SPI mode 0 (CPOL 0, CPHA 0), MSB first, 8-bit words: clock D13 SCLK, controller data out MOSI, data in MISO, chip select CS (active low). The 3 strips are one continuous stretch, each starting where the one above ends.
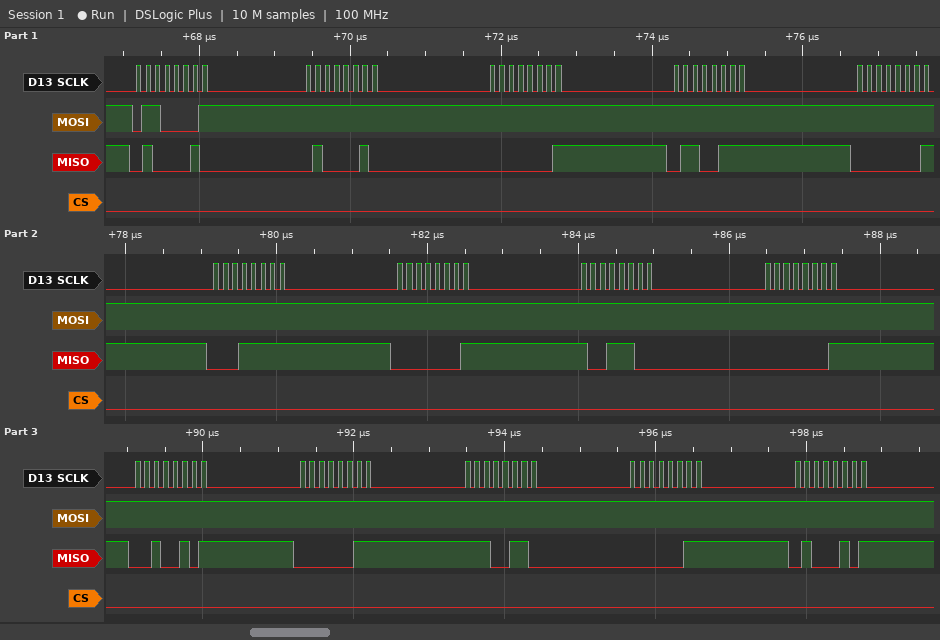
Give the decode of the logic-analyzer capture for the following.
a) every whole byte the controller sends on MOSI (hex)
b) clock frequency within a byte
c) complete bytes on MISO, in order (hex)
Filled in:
61 FF FF FF FF FF FF FF FF FF FF FF FF FF
8 MHz
42 42 01 67 01 1F 01 9C 01 25 03 E6 03 45
